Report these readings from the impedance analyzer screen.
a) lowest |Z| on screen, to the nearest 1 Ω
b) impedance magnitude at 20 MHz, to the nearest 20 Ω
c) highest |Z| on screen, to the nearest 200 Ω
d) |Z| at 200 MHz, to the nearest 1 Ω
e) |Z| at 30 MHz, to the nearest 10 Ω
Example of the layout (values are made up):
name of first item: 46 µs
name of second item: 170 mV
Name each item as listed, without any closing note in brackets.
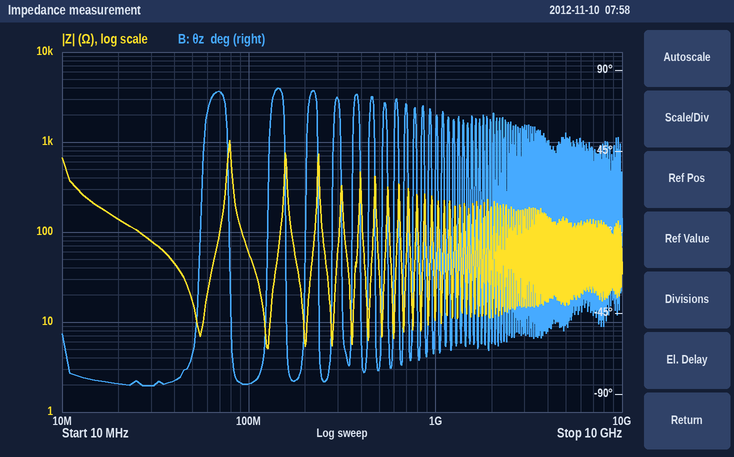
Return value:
lowest |Z| on screen, to the nearest 1 Ω: 5 Ω
impedance magnitude at 20 MHz, to the nearest 20 Ω: 140 Ω
highest |Z| on screen, to the nearest 200 Ω: 1.0 kΩ
|Z| at 200 MHz, to the nearest 1 Ω: 6 Ω
|Z| at 30 MHz, to the nearest 10 Ω: 80 Ω
